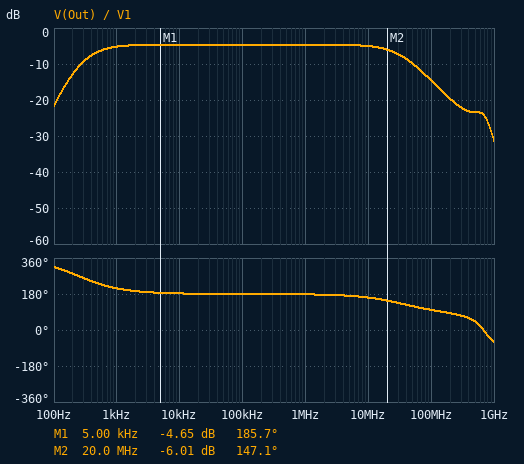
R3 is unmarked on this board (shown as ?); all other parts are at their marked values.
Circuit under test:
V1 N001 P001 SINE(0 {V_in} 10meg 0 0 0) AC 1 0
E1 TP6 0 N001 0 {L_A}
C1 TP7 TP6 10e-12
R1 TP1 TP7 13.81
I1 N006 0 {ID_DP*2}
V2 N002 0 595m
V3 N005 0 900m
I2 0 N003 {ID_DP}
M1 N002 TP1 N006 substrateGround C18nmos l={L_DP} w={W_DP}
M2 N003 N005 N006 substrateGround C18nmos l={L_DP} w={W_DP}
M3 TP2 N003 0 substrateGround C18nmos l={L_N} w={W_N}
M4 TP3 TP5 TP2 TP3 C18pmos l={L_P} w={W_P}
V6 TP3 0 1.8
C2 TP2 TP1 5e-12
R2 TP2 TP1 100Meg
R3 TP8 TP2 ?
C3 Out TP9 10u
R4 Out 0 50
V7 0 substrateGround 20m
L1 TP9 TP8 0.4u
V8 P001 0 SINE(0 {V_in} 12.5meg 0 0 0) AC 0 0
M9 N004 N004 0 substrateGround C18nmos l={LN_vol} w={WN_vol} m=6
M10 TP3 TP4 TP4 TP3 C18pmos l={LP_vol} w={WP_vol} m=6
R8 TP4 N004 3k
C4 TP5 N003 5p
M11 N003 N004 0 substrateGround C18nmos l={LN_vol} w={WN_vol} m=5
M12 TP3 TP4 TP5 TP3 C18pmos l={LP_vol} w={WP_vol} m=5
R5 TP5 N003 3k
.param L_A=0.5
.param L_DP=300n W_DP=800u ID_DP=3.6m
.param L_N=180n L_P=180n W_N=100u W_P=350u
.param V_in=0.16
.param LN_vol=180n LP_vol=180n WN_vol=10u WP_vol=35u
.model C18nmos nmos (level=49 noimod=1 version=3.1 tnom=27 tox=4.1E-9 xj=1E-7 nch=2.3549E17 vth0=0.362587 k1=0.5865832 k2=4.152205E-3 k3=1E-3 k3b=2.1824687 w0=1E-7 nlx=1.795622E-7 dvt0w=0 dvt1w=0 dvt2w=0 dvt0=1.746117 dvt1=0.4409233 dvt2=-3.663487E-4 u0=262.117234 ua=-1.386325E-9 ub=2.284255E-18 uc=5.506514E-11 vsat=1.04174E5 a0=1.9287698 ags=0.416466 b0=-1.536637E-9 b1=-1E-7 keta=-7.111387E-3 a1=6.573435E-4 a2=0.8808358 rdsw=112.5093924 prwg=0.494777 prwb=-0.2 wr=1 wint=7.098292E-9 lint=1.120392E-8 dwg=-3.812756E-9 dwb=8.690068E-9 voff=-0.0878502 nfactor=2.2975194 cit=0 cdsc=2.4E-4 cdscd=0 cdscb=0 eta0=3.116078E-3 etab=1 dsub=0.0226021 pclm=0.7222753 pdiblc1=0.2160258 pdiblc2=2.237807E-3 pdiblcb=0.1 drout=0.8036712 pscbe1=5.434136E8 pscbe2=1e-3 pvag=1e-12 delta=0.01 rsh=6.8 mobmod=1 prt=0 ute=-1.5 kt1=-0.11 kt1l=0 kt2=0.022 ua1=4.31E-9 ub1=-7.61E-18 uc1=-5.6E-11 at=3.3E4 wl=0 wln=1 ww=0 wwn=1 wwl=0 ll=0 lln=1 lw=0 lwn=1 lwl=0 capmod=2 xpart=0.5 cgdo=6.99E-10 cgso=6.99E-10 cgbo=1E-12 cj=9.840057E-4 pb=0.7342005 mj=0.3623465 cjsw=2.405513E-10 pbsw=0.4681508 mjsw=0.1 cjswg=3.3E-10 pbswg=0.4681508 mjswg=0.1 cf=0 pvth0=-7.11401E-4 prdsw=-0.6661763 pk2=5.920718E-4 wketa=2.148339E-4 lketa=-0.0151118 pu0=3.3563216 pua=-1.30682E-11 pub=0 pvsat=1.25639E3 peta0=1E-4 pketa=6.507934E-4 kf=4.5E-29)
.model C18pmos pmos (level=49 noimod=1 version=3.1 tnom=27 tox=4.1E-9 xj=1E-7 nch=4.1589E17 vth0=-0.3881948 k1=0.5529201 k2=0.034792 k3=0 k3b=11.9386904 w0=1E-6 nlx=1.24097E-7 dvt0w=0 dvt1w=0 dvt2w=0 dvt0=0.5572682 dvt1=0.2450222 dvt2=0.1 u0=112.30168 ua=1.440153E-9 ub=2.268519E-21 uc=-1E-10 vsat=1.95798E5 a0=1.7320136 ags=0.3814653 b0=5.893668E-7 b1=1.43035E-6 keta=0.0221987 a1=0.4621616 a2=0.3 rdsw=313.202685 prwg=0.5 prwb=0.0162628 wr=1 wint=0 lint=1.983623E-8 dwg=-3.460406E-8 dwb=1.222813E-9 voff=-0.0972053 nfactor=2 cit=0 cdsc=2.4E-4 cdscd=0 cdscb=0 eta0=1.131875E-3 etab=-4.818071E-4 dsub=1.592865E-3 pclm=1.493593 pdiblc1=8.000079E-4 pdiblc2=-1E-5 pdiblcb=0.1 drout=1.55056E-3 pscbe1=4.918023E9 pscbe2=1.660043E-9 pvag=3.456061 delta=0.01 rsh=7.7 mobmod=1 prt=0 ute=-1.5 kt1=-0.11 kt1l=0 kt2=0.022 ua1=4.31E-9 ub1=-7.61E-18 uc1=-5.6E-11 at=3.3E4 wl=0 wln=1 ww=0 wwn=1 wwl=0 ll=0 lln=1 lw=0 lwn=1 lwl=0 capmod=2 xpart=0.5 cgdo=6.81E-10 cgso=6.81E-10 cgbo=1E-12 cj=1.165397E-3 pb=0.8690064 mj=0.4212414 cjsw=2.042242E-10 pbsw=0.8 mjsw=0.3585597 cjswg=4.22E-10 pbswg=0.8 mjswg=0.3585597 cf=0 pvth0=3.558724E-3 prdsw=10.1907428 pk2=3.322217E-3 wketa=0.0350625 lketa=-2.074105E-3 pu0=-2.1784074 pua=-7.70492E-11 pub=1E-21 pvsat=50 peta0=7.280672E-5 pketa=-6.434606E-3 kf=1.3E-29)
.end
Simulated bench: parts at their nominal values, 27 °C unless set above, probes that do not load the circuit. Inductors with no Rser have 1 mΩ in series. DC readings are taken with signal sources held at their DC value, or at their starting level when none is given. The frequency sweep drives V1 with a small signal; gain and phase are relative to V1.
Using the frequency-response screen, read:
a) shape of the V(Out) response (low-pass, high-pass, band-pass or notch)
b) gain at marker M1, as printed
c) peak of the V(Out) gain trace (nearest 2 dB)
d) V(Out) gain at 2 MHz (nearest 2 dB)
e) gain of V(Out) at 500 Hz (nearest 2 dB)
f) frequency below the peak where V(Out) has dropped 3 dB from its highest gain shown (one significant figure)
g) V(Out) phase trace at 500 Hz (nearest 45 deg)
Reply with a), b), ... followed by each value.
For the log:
a) band-pass
b) -4.65 dB
c) -4 dB
d) -4 dB
e) -6 dB
f) 400 Hz
g) 225 deg
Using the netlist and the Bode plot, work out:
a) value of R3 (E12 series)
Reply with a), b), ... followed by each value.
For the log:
a) 33 Ω
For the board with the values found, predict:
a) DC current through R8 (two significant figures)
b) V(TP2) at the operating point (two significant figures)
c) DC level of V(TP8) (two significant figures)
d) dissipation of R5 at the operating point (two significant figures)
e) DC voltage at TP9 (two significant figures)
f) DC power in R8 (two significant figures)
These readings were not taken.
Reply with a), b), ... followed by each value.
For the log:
a) 240 µA
b) 900 mV
c) 900 mV
d) 120 µW
e) 900 mV
f) 170 µW
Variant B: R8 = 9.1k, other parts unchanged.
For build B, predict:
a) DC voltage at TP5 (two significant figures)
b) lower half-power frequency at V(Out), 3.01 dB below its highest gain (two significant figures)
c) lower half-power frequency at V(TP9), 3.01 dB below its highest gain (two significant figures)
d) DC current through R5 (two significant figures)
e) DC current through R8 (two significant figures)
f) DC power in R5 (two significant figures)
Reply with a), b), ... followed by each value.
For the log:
a) 1.0 V
b) 400 Hz
c) 190 Hz
d) 80 µA
e) 89 µA
f) 19 µW
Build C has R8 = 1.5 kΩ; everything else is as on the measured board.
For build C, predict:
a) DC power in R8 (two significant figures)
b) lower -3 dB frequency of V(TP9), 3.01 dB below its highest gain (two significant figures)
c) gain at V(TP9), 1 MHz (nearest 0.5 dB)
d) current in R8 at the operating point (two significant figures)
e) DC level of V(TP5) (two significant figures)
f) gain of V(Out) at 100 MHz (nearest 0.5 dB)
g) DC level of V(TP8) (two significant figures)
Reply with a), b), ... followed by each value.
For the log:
a) 280 µW
b) 120 MHz
c) -24.0 dB
d) 430 µA
e) 1.4 V
f) -17.5 dB
g) 890 mV
